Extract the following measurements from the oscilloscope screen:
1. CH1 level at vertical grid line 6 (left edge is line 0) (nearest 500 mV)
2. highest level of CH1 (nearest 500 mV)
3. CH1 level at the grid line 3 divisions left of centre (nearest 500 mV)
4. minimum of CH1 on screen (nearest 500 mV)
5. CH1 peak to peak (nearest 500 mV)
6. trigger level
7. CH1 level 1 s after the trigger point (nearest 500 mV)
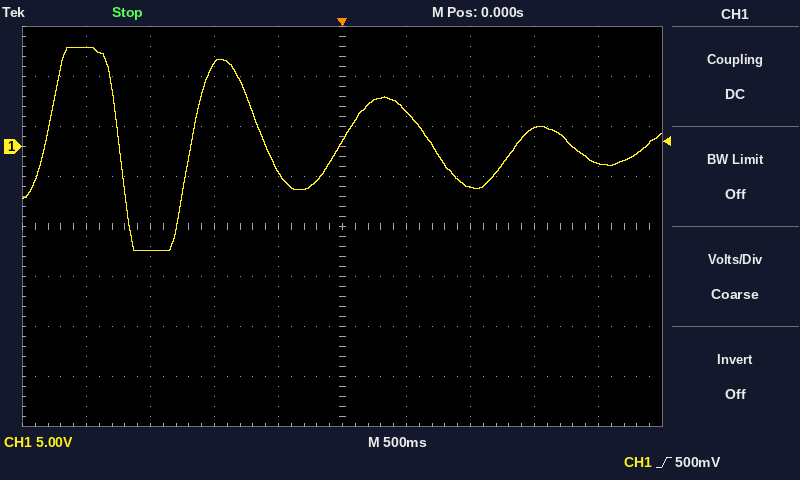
3.5 V
10.0 V
-10.5 V
-10.5 V
20.5 V
500 mV
-4.0 V
